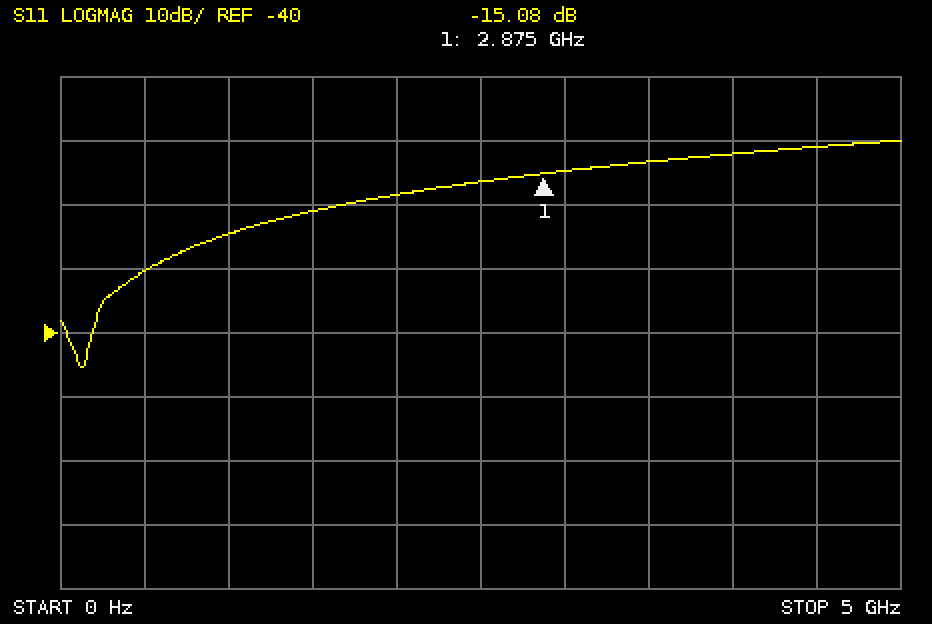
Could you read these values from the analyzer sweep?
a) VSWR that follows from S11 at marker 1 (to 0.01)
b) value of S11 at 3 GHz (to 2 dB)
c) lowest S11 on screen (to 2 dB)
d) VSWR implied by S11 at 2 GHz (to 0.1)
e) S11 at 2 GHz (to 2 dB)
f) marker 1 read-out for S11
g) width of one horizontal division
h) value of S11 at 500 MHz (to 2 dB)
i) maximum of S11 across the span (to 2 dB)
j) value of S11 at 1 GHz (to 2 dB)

1.43
-14 dB
-46 dB
1.3
-18 dB
-15.08 dB
500 MHz
-30 dB
-10 dB
-24 dB
